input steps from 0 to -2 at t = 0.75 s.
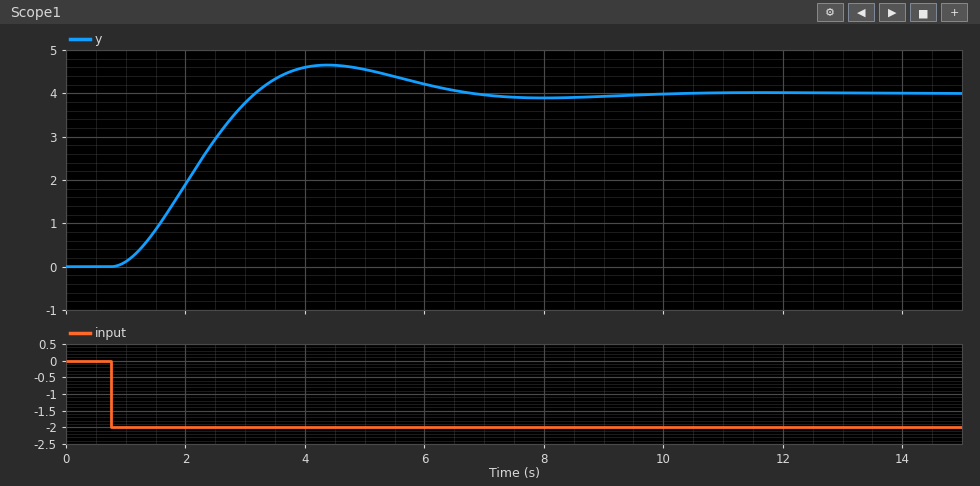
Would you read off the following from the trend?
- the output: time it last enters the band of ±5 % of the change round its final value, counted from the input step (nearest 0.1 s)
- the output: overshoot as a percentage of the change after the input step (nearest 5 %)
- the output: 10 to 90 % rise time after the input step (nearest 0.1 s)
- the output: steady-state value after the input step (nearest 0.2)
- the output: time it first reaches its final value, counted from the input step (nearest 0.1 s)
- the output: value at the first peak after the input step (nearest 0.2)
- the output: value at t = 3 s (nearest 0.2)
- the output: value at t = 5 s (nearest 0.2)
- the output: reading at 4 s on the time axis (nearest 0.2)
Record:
5.3 s
15 %
1.6 s
4.0
2.4 s
4.6
3.8
4.6
4.6
